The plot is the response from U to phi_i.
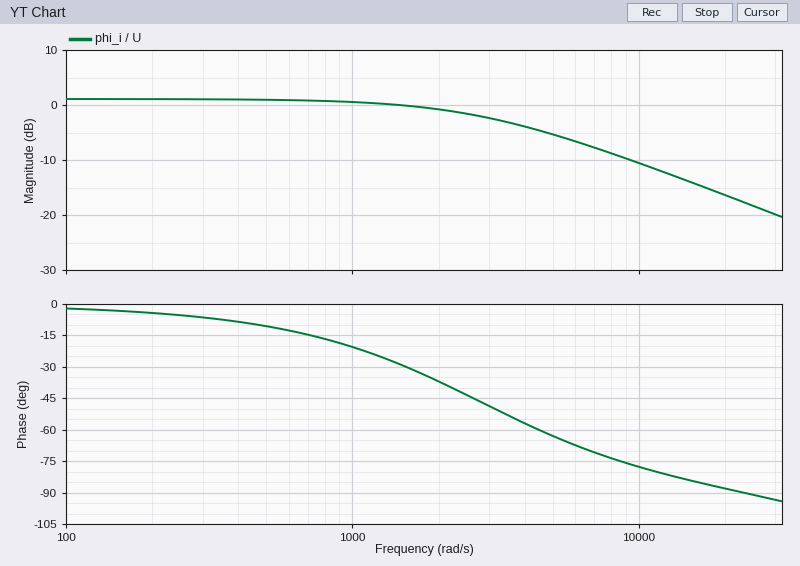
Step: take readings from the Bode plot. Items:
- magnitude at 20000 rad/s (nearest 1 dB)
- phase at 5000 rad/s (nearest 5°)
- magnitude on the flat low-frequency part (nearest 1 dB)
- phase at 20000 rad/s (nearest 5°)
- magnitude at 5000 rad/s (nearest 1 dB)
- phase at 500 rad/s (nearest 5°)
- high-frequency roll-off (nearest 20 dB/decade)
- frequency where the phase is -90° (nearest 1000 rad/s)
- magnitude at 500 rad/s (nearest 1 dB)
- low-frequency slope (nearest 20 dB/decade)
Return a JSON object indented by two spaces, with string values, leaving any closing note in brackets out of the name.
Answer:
{
  "magnitude at 20000 rad/s": "-16 dB",
  "phase at 5000 rad/s": "-65°",
  "magnitude on the flat low-frequency part": "1 dB",
  "phase at 20000 rad/s": "-90°",
  "magnitude at 5000 rad/s": "-5 dB",
  "phase at 500 rad/s": "-10°",
  "high-frequency roll-off": "-20 dB/decade",
  "frequency where the phase is -90°": "23000 rad/s",
  "magnitude at 500 rad/s": "1 dB",
  "low-frequency slope": "0 dB/decade"
}
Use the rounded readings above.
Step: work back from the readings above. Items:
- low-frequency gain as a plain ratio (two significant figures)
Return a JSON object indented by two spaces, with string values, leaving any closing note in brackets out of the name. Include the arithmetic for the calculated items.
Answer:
{
  "low-frequency gain as a plain ratio": "10^(1 / 20) = 1.1"
}
